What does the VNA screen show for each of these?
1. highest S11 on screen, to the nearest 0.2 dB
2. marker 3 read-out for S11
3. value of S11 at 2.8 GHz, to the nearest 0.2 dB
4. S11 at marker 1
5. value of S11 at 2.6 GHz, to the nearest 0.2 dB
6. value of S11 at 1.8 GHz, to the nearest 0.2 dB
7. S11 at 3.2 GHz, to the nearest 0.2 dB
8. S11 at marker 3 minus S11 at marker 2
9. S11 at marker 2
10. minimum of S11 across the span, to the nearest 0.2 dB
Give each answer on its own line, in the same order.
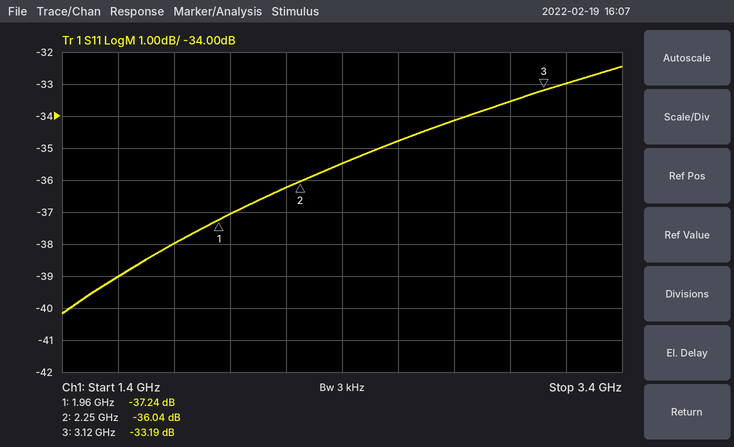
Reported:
-32.4 dB
-33.19 dB
-34.2 dB
-37.24 dB
-34.8 dB
-38.0 dB
-33.0 dB
2.85 dB
-36.04 dB
-40.2 dB
